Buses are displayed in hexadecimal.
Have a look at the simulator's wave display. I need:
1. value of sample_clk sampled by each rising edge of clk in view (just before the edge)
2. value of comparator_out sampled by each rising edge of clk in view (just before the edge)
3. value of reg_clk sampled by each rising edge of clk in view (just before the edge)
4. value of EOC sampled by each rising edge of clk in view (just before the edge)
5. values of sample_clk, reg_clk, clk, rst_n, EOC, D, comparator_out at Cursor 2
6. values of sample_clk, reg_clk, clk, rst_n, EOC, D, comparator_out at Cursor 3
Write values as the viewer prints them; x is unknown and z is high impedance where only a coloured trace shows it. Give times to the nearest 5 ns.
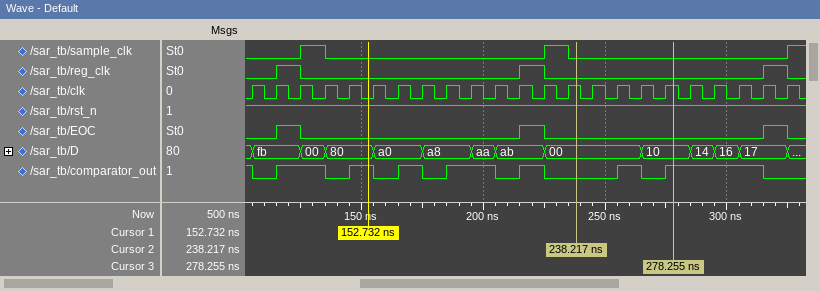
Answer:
0 0 0 1 0 0 0 0 0 0 0 0 0 1 0 0 0 0 0 0 0 0 0
1 0 1 1 0 1 0 1 0 1 1 0 1 0 0 0 1 0 1 1 1 1 0
0 0 1 0 0 0 0 0 0 0 0 0 1 0 0 0 0 0 0 0 0 0 1
0 0 1 0 0 0 0 0 0 0 0 0 1 0 0 0 0 0 0 0 0 0 1
sample_clk=0, reg_clk=0, clk=1, rst_n=1, EOC=0, D=00, comparator_out=0
sample_clk=0, reg_clk=0, clk=1, rst_n=1, EOC=0, D=10, comparator_out=1
